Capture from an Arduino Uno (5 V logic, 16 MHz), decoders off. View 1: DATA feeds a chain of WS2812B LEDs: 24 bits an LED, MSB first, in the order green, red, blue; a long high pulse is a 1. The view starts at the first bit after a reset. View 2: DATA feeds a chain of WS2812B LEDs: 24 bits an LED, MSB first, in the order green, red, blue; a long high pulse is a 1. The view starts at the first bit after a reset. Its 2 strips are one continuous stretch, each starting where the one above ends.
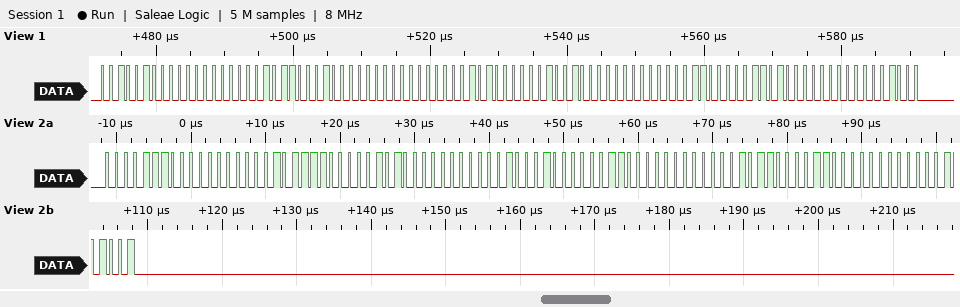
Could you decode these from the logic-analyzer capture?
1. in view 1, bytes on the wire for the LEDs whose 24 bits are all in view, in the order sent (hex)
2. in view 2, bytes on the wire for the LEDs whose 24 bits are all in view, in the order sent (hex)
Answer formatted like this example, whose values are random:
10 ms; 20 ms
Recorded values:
24 00 16 20 00 14 09 00 06 0D 00 08; 0E 00 2F 05 00 11 03 00 0B 0C 00 29
